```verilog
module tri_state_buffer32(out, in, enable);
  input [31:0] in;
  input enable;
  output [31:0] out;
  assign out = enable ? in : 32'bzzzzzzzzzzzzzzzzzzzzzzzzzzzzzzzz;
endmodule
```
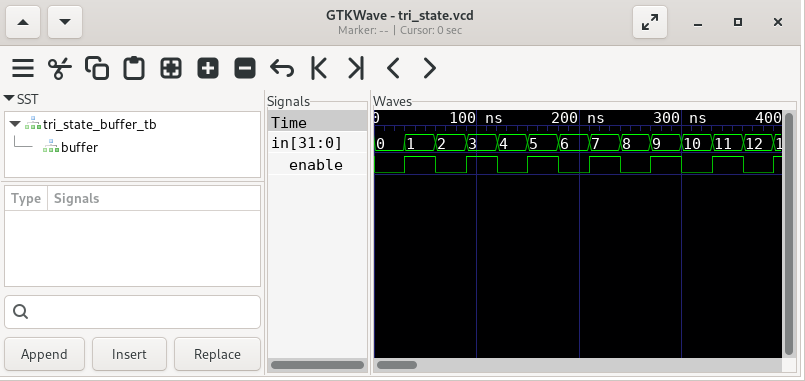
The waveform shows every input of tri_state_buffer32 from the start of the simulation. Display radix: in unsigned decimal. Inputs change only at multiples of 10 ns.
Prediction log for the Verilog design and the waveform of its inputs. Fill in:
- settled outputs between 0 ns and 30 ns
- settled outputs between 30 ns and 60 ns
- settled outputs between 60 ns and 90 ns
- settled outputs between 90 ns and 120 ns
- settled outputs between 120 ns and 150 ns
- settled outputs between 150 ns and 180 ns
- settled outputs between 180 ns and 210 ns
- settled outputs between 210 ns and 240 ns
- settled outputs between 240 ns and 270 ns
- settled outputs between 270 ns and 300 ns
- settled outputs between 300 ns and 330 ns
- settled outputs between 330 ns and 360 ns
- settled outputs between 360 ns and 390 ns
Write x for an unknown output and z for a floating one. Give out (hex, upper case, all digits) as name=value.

out=z
out=00000001
out=z
out=00000003
out=z
out=00000005
out=z
out=00000007
out=z
out=00000009
out=z
out=0000000B
out=z
